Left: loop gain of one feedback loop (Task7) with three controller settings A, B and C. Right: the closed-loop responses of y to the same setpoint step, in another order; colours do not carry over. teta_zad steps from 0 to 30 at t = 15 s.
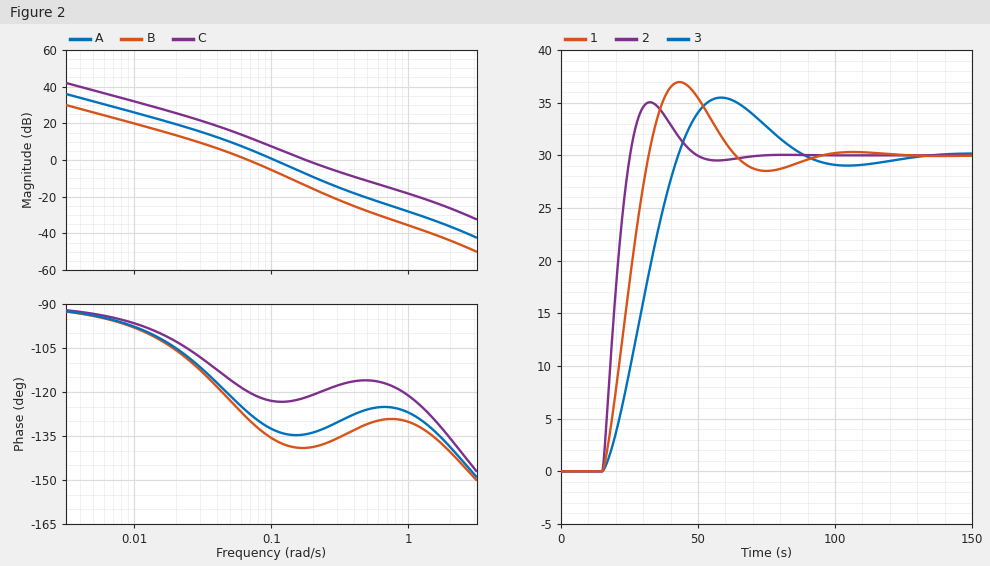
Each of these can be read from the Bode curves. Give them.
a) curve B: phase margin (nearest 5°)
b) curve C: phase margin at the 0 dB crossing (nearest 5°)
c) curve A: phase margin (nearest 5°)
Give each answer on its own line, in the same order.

50°
60°
45°
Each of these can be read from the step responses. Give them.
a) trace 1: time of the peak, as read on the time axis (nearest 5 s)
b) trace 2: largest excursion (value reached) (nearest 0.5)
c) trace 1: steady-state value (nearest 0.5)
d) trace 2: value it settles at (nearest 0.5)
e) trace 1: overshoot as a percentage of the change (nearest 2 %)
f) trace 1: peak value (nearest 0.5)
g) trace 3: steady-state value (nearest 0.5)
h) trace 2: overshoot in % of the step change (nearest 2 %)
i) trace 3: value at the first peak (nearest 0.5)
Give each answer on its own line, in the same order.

45 s
35.0
30.0
30.0
24 %
37.0
30.0
16 %
35.5
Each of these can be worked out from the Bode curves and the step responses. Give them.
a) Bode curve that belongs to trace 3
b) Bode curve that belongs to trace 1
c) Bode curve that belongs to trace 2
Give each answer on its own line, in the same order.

B
A
C
